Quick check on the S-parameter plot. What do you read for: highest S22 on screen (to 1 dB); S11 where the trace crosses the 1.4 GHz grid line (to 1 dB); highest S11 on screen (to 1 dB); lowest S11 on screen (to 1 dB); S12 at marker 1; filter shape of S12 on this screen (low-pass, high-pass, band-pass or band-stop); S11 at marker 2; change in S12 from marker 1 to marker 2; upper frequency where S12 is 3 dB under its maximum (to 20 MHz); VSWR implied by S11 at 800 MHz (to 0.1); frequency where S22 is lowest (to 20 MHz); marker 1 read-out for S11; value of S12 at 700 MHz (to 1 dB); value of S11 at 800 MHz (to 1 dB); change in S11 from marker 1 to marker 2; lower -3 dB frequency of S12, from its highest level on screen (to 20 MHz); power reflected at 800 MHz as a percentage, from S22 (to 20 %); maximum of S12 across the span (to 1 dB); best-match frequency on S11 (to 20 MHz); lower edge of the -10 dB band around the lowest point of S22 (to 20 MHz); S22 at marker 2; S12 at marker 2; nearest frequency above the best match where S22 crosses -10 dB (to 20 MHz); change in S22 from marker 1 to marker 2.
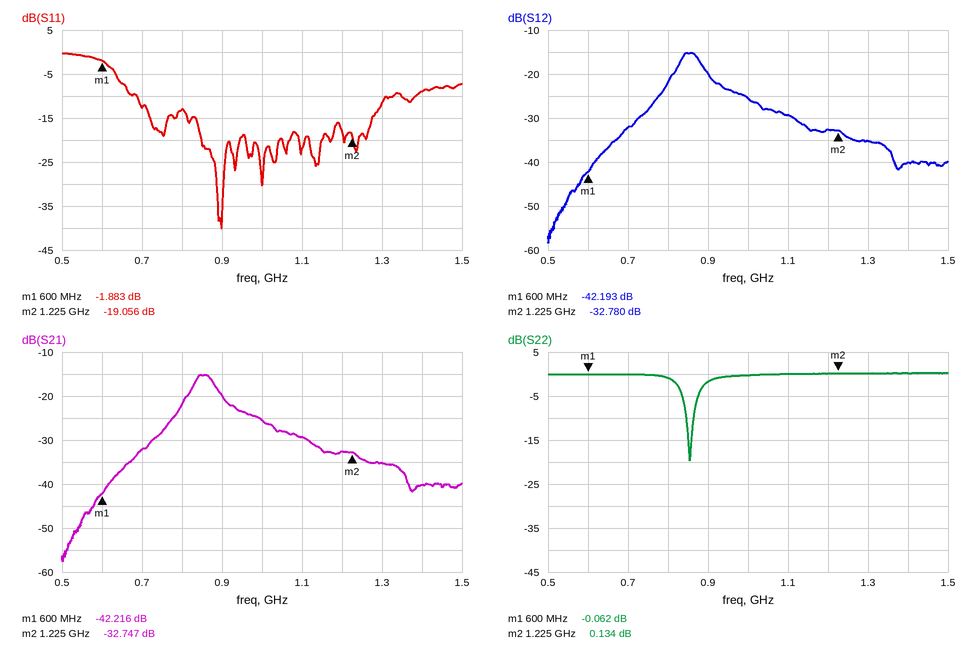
0 dB
-9 dB
0 dB
-40 dB
-42.193 dB
band-pass
-19.056 dB
9.413 dB
880 MHz
1.6
860 MHz
-1.883 dB
-32 dB
-13 dB
-17.173 dB
820 MHz
80 %
-15 dB
900 MHz
840 MHz
0.134 dB
-32.780 dB
860 MHz
0.196 dB
